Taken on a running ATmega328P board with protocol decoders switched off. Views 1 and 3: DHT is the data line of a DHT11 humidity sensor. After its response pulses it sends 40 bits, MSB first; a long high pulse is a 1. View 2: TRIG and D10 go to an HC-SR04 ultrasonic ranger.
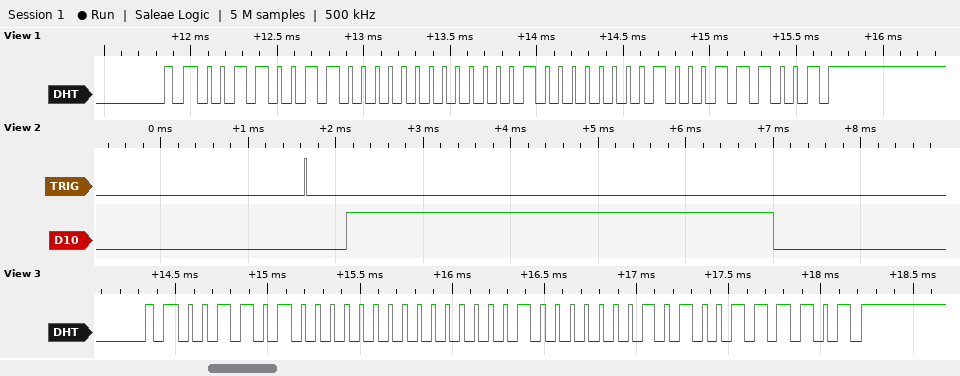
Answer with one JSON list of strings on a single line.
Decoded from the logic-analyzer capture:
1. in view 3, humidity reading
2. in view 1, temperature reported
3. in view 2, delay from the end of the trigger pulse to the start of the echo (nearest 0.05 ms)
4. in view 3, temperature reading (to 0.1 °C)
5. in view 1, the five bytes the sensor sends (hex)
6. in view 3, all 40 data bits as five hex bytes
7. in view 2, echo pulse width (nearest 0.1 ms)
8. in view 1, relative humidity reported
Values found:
["52 %", "4.2 °C", "0.45 ms", "4.5 °C", "33 00 04 02 39", "34 00 04 05 3D", "4.9 ms", "51 %"]
